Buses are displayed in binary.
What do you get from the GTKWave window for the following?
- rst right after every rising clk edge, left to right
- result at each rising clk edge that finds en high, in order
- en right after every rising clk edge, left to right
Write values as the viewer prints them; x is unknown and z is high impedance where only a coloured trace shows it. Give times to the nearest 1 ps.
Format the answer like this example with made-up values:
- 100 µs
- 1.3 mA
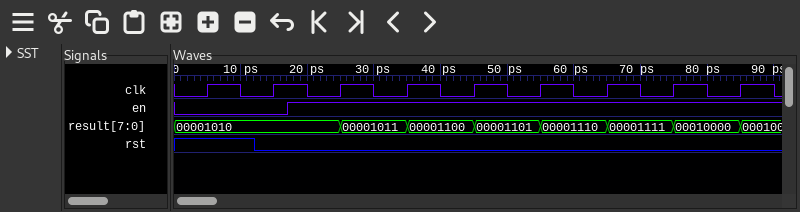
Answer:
- 1 0 0 0 0 0 0 0 0
- 00001010, 00001011, 00001100, 00001101, 00001110, 00001111, 00010000
- 0 0 1 1 1 1 1 1 1
